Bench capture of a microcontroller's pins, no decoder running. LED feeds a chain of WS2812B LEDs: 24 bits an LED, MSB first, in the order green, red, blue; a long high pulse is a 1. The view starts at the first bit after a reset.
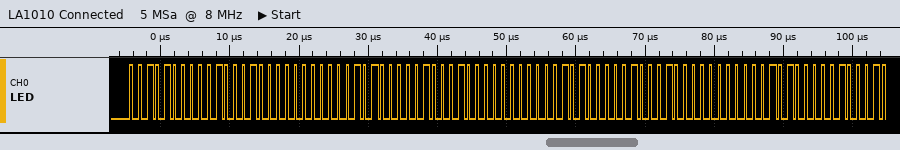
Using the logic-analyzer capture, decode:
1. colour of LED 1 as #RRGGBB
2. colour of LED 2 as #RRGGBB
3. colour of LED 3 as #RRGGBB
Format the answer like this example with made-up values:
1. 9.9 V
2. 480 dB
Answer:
1. #222800
2. #222800
3. #222800
